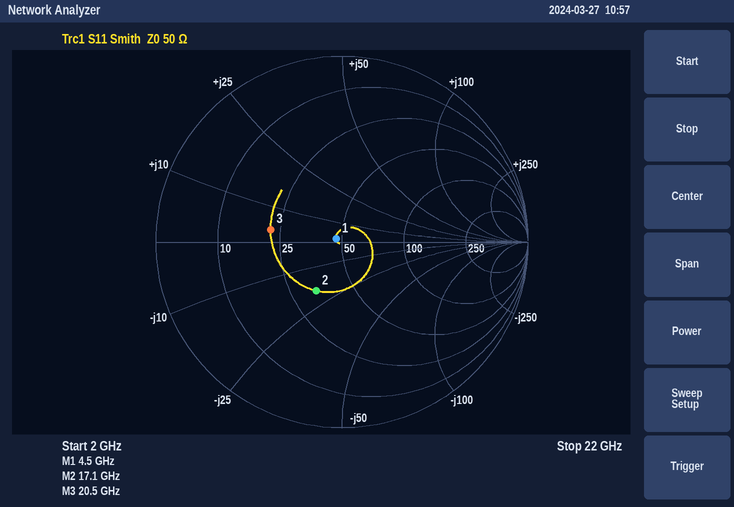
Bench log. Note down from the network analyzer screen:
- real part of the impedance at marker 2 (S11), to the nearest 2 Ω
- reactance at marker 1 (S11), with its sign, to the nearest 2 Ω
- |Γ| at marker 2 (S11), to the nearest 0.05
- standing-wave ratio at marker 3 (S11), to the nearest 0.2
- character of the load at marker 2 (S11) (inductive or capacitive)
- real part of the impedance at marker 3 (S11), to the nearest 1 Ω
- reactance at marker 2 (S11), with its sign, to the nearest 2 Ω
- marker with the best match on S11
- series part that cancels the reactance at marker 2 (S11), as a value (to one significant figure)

34 Ω
+2 Ω
0.30
2.2
capacitive
22 Ω
-20 Ω
marker 1
200 pH
